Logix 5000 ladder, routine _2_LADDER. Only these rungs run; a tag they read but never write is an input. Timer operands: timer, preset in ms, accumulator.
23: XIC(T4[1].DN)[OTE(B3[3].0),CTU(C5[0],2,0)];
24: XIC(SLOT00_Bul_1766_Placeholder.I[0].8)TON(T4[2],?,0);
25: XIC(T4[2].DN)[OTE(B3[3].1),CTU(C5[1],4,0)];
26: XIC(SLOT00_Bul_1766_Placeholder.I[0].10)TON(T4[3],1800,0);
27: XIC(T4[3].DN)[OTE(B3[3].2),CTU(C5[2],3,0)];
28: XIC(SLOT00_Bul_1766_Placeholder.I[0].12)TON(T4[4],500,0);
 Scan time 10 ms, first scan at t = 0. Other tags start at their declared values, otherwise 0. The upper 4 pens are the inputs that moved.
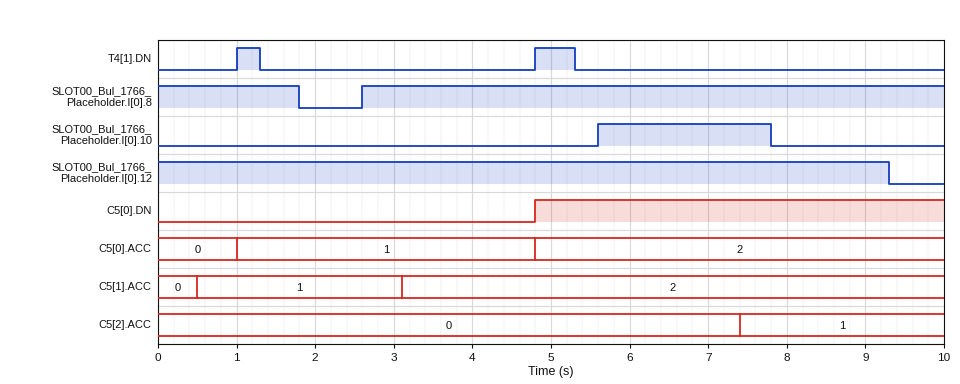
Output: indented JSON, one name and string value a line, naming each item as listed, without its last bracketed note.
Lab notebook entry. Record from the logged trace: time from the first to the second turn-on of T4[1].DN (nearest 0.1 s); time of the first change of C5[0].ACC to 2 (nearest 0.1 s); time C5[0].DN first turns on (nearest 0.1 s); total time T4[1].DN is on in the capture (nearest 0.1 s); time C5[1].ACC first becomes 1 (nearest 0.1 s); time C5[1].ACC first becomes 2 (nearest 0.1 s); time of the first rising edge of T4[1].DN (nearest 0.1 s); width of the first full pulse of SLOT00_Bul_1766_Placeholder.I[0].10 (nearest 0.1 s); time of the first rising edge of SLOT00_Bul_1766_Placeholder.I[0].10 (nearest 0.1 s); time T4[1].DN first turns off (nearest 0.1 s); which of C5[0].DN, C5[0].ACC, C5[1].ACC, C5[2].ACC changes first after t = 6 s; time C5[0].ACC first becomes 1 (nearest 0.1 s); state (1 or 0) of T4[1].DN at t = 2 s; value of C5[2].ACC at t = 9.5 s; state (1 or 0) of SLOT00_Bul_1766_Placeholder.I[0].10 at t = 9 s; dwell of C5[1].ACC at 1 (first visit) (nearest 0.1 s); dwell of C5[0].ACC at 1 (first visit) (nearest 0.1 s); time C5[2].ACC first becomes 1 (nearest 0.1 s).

{
  "time from the first to the second turn-on of T4[1].DN": "3.8 s",
  "time of the first change of C5[0].ACC to 2": "4.8 s",
  "time C5[0].DN first turns on": "4.8 s",
  "total time T4[1].DN is on in the capture": "0.8 s",
  "time C5[1].ACC first becomes 1": "0.5 s",
  "time C5[1].ACC first becomes 2": "3.1 s",
  "time of the first rising edge of T4[1].DN": "1.0 s",
  "width of the first full pulse of SLOT00_Bul_1766_Placeholder.I[0].10": "2.2 s",
  "time of the first rising edge of SLOT00_Bul_1766_Placeholder.I[0].10": "5.6 s",
  "time T4[1].DN first turns off": "1.3 s",
  "which of C5[0].DN, C5[0].ACC, C5[1].ACC, C5[2].ACC changes first after t = 6 s": "C5[2].ACC",
  "time C5[0].ACC first becomes 1": "1.0 s",
  "state (1 or 0) of T4[1].DN at t = 2 s": "0",
  "value of C5[2].ACC at t = 9.5 s": "1",
  "state (1 or 0) of SLOT00_Bul_1766_Placeholder.I[0].10 at t = 9 s": "0",
  "dwell of C5[1].ACC at 1 (first visit)": "2.6 s",
  "dwell of C5[0].ACC at 1 (first visit)": "3.8 s",
  "time C5[2].ACC first becomes 1": "7.4 s"
}
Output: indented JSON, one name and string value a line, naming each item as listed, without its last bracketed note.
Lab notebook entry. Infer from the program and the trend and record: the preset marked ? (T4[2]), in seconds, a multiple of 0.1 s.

{
  "the preset marked ? (T4[2]), in seconds, a multiple of 0.1 s": "0.5 s"
}
